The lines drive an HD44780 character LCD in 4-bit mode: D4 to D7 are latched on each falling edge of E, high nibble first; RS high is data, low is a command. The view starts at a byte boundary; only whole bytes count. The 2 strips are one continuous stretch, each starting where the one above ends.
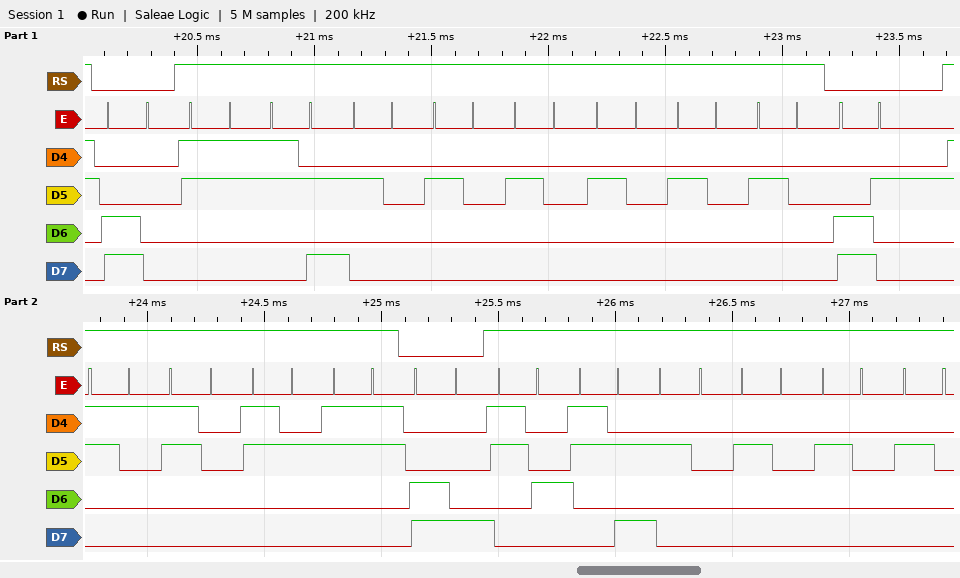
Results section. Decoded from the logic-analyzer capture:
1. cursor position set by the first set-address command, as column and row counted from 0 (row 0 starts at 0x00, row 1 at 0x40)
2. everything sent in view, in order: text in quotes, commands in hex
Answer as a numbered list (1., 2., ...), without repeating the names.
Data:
1. column 0, row 1
2. 0xC0 "3:      " 0xC2 "1023" 0xC8 "4:    "
